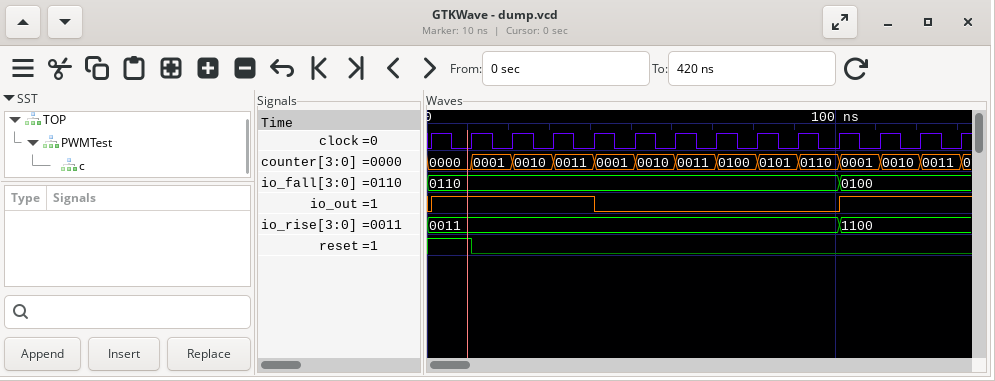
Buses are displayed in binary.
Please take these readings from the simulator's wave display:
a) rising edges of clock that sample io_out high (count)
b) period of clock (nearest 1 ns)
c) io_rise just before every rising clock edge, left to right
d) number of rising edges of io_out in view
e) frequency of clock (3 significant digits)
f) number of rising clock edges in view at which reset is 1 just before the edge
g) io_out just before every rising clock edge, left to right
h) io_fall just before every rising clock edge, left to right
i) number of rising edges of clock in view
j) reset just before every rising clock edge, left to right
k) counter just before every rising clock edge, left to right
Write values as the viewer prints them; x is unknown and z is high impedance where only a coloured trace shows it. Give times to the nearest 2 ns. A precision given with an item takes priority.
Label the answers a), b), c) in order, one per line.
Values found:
a) 7
b) 10 ns
c) 0011, 0011, 0011, 0011, 0011, 0011, 0011, 0011, 0011, 0011, 0011, 1100, 1100, 1100
d) 2
e) 100 MHz
f) 2
g) 0 1 1 1 1 0 0 0 0 0 0 1 1 1
h) 0110, 0110, 0110, 0110, 0110, 0110, 0110, 0110, 0110, 0110, 0110, 0100, 0100, 0100
i) 14
j) 1 1 0 0 0 0 0 0 0 0 0 0 0 0
k) 0000, 0000, 0001, 0010, 0011, 0001, 0010, 0011, 0100, 0101, 0110, 0001, 0010, 0011
